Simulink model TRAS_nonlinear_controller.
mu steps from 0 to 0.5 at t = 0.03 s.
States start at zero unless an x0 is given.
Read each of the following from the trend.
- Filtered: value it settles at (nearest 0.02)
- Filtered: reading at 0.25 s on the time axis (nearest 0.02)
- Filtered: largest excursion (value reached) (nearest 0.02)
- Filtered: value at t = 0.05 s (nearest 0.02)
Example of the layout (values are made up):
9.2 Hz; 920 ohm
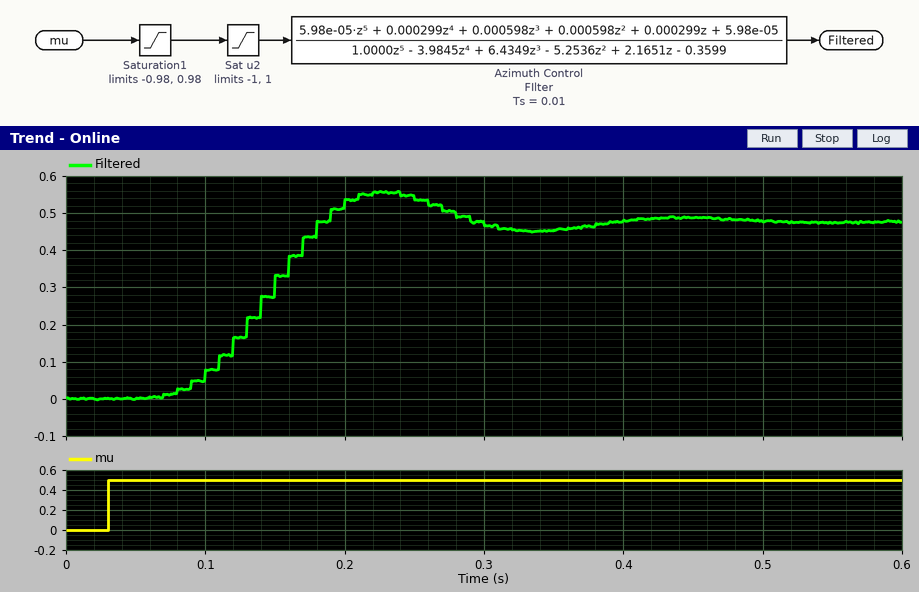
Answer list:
0.48; 0.54; 0.56; 0.00
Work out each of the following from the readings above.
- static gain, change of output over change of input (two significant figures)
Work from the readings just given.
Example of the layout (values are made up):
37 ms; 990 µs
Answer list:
0.96
